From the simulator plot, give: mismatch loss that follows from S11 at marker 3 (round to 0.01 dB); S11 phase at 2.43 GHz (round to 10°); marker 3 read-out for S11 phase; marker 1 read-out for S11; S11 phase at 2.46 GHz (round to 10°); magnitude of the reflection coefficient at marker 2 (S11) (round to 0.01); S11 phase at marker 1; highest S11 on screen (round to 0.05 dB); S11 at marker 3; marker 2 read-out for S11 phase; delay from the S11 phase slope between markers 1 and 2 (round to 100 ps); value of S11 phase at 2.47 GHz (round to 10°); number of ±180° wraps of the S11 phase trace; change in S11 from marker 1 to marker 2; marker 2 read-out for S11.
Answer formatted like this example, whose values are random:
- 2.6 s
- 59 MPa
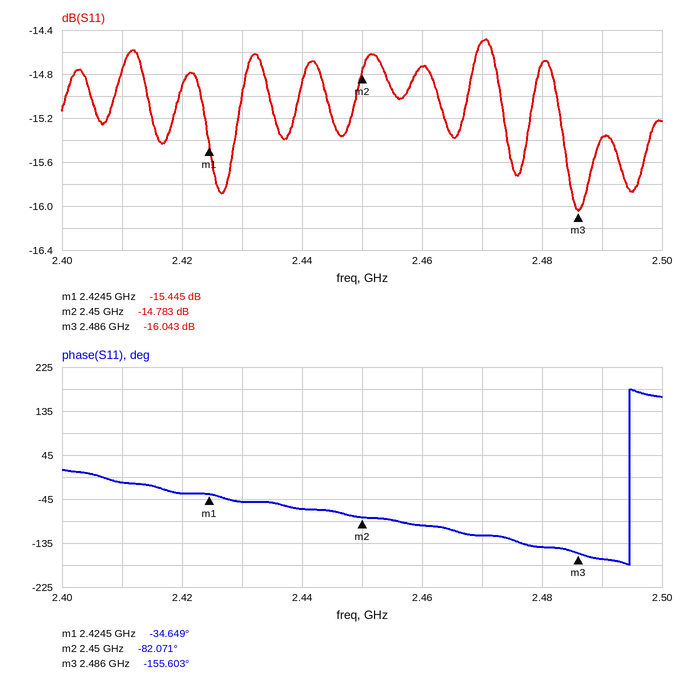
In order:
- 0.11 dB
- -50°
- -155.603°
- -15.445 dB
- -100°
- 0.18
- -34.649°
- -14.50 dB
- -16.043 dB
- -82.071°
- 5.2 ns
- -120°
- 1
- 0.662 dB
- -14.783 dB
